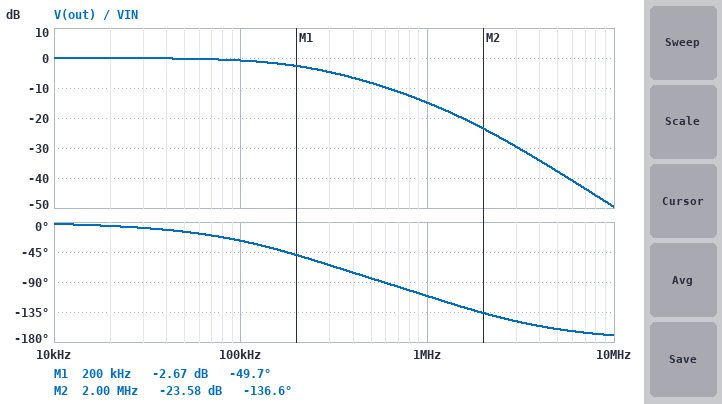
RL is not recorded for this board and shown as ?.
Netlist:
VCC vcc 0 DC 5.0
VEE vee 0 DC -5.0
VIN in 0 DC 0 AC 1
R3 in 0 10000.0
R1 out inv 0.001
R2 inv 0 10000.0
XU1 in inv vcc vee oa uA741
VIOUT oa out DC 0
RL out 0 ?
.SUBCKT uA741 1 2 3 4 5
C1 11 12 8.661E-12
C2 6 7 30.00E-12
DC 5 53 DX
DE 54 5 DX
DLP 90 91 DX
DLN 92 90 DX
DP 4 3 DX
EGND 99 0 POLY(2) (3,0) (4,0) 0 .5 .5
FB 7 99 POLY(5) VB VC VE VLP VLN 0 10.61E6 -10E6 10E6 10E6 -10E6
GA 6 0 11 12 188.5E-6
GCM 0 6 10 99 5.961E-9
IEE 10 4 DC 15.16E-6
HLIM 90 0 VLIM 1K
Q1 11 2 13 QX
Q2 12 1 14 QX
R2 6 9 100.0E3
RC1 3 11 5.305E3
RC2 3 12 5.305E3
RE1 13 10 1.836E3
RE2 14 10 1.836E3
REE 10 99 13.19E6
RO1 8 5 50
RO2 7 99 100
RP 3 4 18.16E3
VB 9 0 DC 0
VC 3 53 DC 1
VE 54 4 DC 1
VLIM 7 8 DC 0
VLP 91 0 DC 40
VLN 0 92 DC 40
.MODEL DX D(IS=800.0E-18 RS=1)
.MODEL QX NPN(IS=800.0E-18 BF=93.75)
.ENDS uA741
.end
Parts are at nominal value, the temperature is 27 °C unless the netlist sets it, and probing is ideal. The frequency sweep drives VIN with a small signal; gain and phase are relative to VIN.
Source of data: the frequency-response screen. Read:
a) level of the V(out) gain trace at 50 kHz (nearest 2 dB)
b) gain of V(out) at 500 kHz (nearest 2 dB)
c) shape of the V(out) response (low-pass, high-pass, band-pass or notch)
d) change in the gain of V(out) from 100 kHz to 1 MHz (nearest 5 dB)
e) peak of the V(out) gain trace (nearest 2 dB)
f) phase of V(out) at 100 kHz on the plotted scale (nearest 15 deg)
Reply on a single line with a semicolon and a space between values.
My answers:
0 dB; -8 dB; low-pass; -15 dB; 0 dB; -30 deg
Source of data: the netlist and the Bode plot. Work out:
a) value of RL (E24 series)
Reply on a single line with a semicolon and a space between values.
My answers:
12 Ω
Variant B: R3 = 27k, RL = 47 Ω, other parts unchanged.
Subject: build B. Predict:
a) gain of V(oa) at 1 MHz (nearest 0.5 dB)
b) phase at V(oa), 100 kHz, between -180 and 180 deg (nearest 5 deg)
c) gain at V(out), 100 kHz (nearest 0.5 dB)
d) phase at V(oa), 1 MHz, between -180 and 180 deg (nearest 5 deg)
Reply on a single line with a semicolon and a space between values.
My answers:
-6.5 dB; -10 deg; 0 dB; -95 deg
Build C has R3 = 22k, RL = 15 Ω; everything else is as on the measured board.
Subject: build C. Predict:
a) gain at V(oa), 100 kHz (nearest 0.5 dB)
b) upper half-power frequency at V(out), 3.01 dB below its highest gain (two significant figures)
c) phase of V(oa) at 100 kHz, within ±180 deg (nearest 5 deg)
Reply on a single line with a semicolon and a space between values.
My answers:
-0.5 dB; 260 kHz; -25 deg
